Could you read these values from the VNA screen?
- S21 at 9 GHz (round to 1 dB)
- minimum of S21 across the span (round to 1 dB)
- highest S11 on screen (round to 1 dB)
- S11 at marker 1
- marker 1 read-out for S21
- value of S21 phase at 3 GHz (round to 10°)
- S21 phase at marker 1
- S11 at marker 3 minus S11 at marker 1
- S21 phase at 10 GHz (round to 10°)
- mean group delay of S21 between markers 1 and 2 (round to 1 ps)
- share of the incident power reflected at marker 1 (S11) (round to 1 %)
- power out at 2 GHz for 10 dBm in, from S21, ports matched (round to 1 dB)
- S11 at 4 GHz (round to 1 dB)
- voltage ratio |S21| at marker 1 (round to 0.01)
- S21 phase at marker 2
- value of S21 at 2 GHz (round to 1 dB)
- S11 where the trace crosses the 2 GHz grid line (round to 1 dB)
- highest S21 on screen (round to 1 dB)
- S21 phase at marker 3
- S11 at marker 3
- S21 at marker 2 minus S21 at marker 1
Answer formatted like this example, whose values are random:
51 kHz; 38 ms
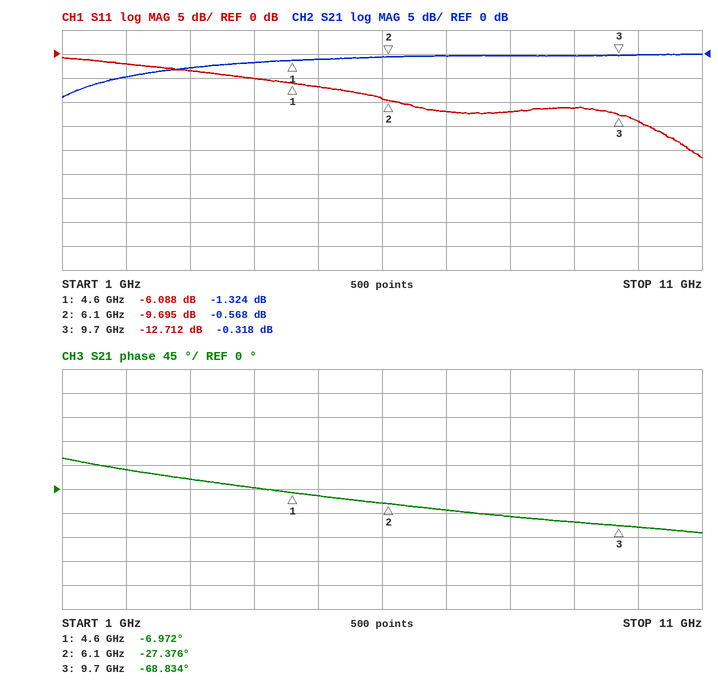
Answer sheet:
0 dB; -9 dB; -1 dB; -6.088 dB; -1.324 dB; 20°; -6.972°; -6.624 dB; -70°; 38 ps; 25 %; 5 dBm; -5 dB; 0.86; -27.376°; -5 dB; -2 dB; 0 dB; -68.834°; -12.712 dB; 0.756 dB
